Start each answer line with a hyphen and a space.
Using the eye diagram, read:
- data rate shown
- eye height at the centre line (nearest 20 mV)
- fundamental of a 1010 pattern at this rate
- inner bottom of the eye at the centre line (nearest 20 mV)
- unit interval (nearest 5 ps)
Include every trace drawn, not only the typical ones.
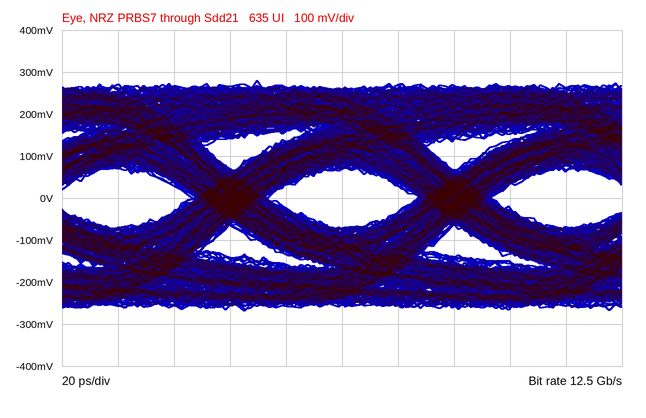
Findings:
- 12.5 Gb/s
- 140 mV
- 6.25 GHz
- -80 mV
- 80 ps
